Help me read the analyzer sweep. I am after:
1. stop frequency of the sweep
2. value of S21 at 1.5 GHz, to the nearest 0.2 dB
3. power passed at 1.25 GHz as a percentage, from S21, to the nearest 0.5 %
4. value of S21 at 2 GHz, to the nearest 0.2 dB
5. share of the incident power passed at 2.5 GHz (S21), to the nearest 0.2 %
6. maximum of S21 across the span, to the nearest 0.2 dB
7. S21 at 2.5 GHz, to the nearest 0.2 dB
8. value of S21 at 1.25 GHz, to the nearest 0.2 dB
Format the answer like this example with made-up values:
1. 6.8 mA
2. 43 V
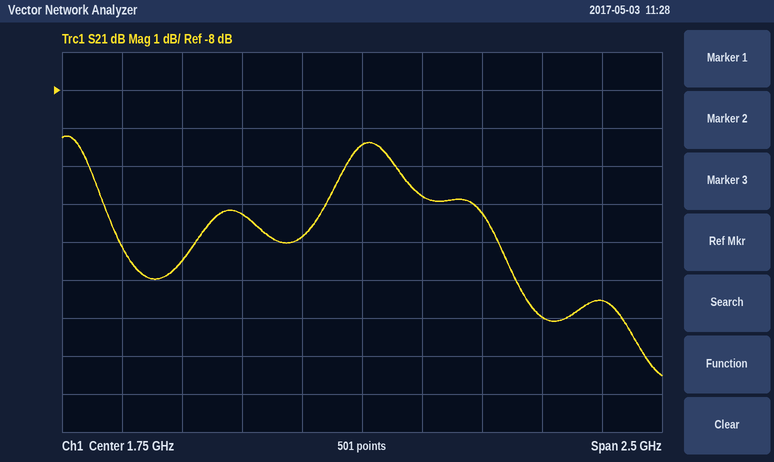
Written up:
1. 3 GHz
2. -11.8 dB
3. 7.5 %
4. -10.8 dB
5. 4.0 %
6. -9.2 dB
7. -14.0 dB
8. -11.2 dB
